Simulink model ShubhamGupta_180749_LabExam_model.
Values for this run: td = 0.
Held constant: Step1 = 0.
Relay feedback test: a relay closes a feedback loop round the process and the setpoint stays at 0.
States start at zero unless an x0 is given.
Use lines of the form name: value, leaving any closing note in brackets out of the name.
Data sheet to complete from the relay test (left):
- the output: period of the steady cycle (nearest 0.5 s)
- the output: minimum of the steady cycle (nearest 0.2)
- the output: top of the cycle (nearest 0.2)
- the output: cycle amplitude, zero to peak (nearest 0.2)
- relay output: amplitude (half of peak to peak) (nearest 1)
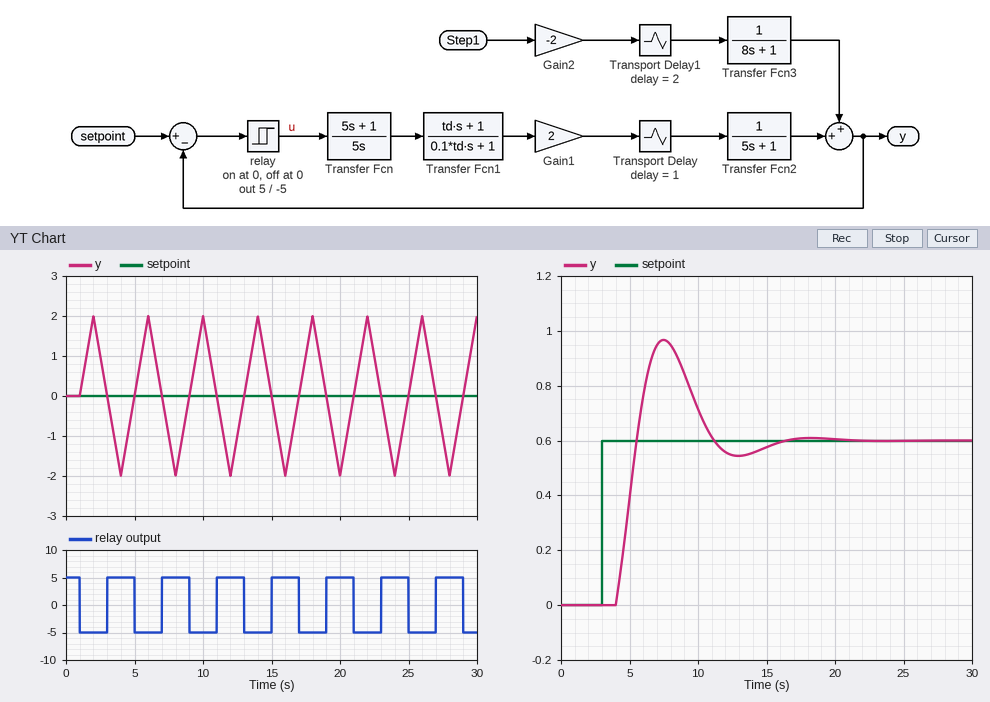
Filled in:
the output: period of the steady cycle: 4.0 s
the output: minimum of the steady cycle: -2.0
the output: top of the cycle: 2.0
the output: cycle amplitude, zero to peak: 2.0
relay output: amplitude (half of peak to peak): 5
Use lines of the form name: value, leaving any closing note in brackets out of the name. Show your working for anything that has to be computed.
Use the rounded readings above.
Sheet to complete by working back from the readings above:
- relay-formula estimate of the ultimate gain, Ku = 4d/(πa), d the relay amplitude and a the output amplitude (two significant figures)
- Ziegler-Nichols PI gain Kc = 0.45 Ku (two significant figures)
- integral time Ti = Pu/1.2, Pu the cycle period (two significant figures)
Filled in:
relay-formula estimate of the ultimate gain, Ku = 4d/(πa), d the relay amplitude and a the output amplitude: 4 × 5 / (π × 2) = 3.2
Ziegler-Nichols PI gain Kc = 0.45 Ku: 0.45 × 3.2 = 1.4
integral time Ti = Pu/1.2, Pu the cycle period: 4 / 1.2 = 3.3 s
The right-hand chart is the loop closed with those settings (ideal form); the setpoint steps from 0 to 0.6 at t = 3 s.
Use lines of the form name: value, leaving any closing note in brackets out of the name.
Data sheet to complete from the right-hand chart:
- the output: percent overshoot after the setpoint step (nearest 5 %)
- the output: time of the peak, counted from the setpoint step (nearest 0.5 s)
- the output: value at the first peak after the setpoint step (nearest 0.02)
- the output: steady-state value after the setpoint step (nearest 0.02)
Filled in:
the output: percent overshoot after the setpoint step: 60 %
the output: time of the peak, counted from the setpoint step: 4.5 s
the output: value at the first peak after the setpoint step: 0.96
the output: steady-state value after the setpoint step: 0.60
